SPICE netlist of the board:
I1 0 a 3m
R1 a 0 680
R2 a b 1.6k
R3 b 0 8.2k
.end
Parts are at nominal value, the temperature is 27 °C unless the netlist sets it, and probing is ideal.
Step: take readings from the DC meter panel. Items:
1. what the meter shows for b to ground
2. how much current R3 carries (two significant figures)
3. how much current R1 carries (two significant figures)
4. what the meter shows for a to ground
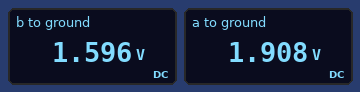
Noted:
1.596 V
190 µA
2.8 mA
1.908 V
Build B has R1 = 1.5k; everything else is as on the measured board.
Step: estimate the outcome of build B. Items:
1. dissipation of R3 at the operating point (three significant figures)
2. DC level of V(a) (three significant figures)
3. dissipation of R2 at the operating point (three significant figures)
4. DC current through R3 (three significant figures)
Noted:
1.30 mW
3.90 V
254 µW
398 µA
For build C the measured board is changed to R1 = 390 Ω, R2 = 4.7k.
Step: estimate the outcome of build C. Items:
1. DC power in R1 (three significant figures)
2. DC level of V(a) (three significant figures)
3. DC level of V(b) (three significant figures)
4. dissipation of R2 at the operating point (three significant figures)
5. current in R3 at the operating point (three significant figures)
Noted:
3.31 mW
1.14 V
722 mV
36.4 µW
88.0 µA
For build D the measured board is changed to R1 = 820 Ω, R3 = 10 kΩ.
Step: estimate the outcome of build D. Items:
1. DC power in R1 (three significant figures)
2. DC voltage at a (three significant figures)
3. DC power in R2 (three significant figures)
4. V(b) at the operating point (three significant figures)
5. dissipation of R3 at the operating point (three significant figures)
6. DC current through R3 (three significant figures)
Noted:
6.44 mW
2.30 V
62.8 µW
1.98 V
392 µW
198 µA
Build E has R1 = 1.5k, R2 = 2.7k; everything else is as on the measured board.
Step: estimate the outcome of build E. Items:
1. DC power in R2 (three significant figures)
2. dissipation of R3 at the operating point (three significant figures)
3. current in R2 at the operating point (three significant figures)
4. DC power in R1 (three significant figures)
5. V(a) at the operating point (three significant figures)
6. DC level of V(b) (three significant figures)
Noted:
356 µW
1.08 mW
363 µA
10.4 mW
3.96 V
2.98 V
